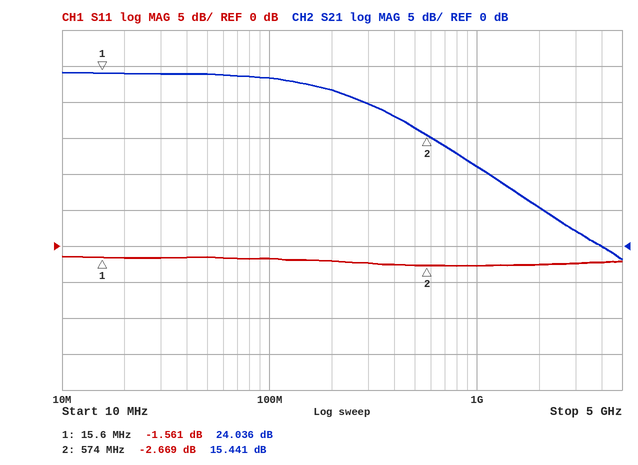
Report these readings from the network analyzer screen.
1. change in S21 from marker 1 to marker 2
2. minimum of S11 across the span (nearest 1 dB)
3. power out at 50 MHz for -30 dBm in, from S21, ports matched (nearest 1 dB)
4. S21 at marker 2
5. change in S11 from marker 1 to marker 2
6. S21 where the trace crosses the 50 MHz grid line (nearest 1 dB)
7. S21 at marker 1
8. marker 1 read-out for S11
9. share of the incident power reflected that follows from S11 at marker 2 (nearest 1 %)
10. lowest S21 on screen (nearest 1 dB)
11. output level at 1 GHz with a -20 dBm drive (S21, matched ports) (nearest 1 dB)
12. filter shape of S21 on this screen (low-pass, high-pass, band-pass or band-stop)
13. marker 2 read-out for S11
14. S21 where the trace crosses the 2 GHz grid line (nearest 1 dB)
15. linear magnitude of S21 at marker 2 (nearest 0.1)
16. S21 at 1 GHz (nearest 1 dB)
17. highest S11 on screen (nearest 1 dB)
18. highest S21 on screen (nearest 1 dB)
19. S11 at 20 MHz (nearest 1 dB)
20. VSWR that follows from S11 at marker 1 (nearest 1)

-8.595 dB
-3 dB
-6 dBm
15.441 dB
-1.108 dB
24 dB
24.036 dB
-1.561 dB
54 %
-2 dB
-9 dBm
low-pass
-2.669 dB
5 dB
5.9
11 dB
-1 dB
24 dB
-2 dB
11
